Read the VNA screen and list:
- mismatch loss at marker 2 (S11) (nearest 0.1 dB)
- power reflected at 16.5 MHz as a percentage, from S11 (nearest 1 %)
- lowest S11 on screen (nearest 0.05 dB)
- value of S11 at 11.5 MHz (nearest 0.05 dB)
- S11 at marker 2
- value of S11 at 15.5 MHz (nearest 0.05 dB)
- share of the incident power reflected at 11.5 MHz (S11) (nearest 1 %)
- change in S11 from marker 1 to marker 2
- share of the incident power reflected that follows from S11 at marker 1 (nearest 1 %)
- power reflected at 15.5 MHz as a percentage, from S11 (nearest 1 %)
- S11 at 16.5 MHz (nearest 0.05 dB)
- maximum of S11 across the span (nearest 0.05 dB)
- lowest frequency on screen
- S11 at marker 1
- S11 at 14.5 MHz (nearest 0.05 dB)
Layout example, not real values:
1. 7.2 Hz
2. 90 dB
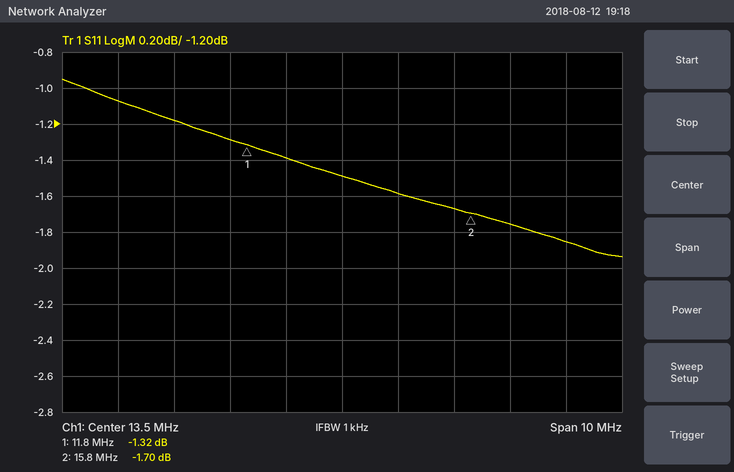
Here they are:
1. 4.9 dB
2. 67 %
3. -1.95 dB
4. -1.30 dB
5. -1.70 dB
6. -1.65 dB
7. 74 %
8. -0.38 dB
9. 74 %
10. 68 %
11. -1.75 dB
12. -0.95 dB
13. 8.5 MHz
14. -1.32 dB
15. -1.60 dB
